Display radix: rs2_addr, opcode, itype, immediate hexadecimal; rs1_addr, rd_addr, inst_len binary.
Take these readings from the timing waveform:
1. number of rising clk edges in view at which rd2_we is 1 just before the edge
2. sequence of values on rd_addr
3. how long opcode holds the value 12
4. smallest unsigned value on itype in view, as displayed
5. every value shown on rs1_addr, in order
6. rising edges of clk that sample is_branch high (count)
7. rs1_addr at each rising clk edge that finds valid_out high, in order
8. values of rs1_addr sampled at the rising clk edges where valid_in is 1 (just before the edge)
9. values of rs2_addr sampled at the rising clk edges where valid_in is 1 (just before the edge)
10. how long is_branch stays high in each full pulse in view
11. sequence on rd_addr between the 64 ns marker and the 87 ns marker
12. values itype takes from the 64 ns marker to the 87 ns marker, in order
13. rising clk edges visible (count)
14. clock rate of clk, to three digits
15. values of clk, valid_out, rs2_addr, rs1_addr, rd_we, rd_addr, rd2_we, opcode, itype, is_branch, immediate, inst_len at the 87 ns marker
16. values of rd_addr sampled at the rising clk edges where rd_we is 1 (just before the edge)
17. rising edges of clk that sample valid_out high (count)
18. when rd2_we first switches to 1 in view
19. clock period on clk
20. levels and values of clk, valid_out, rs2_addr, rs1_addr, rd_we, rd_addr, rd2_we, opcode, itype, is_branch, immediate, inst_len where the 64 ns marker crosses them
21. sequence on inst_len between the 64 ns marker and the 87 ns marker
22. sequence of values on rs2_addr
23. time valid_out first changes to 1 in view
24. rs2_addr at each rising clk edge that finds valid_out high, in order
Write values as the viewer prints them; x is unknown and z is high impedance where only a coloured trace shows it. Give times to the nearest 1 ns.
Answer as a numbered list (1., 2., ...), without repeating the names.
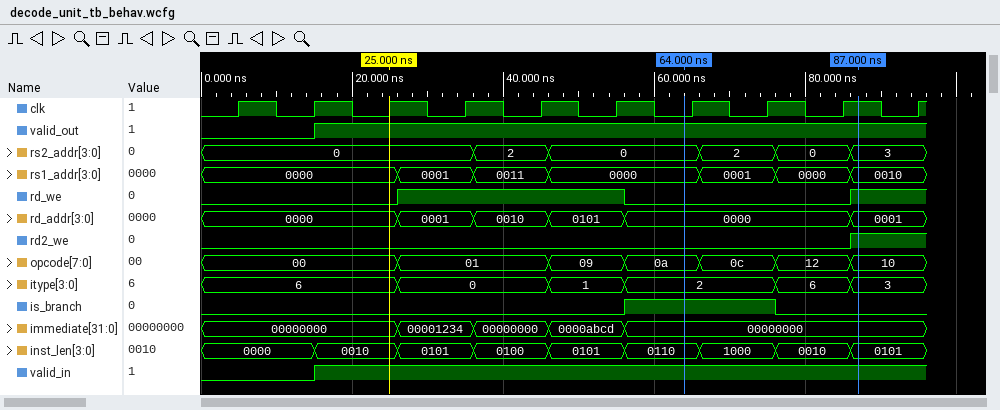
1. 1
2. 0000, 0001, 0010, 0101, 0000, 0001
3. 10 ns
4. 0
5. 0000, 0001, 0011, 0000, 0001, 0000, 0010
6. 2
7. 0000, 0001, 0011, 0000, 0000, 0001, 0000, 0010
8. 0000, 0001, 0011, 0000, 0000, 0001, 0000, 0010
9. 0, 0, 2, 0, 0, 2, 0, 3
10. 20 ns
11. 0000, 0001
12. 2, 6, 3
13. 10
14. 100 MHz
15. clk=1, valid_out=1, rs2_addr=3, rs1_addr=0010, rd_we=1, rd_addr=0001, rd2_we=1, opcode=10, itype=3, is_branch=0, immediate=00000000, inst_len=0101
16. 0001, 0010, 0101, 0001
17. 8
18. 86 ns
19. 10 ns
20. clk=0, valid_out=1, rs2_addr=0, rs1_addr=0000, rd_we=0, rd_addr=0000, rd2_we=0, opcode=0a, itype=2, is_branch=1, immediate=00000000, inst_len=0110
21. 0110, 1000, 0010, 0101
22. 0, 2, 0, 2, 0, 3
23. 15 ns
24. 0, 0, 2, 0, 0, 2, 0, 3
